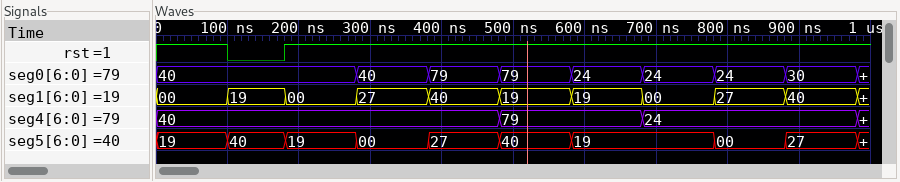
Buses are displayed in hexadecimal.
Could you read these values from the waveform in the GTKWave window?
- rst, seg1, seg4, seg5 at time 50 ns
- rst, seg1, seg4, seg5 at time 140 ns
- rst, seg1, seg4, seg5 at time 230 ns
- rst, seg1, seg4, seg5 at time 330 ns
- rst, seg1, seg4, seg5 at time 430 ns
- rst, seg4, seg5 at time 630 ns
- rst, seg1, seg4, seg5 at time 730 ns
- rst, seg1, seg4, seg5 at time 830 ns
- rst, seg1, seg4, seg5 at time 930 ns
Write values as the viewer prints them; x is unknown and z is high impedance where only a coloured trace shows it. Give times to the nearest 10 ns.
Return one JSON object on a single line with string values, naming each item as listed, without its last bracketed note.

{"rst, seg1, seg4, seg5 at time 50 ns": "rst=1, seg1=00, seg4=40, seg5=19", "rst, seg1, seg4, seg5 at time 140 ns": "rst=0, seg1=19, seg4=40, seg5=40", "rst, seg1, seg4, seg5 at time 230 ns": "rst=1, seg1=00, seg4=40, seg5=19", "rst, seg1, seg4, seg5 at time 330 ns": "rst=1, seg1=27, seg4=40, seg5=00", "rst, seg1, seg4, seg5 at time 430 ns": "rst=1, seg1=40, seg4=40, seg5=27", "rst, seg4, seg5 at time 630 ns": "rst=1, seg4=79, seg5=19", "rst, seg1, seg4, seg5 at time 730 ns": "rst=1, seg1=00, seg4=24, seg5=19", "rst, seg1, seg4, seg5 at time 830 ns": "rst=1, seg1=27, seg4=24, seg5=00", "rst, seg1, seg4, seg5 at time 930 ns": "rst=1, seg1=40, seg4=24, seg5=27"}
